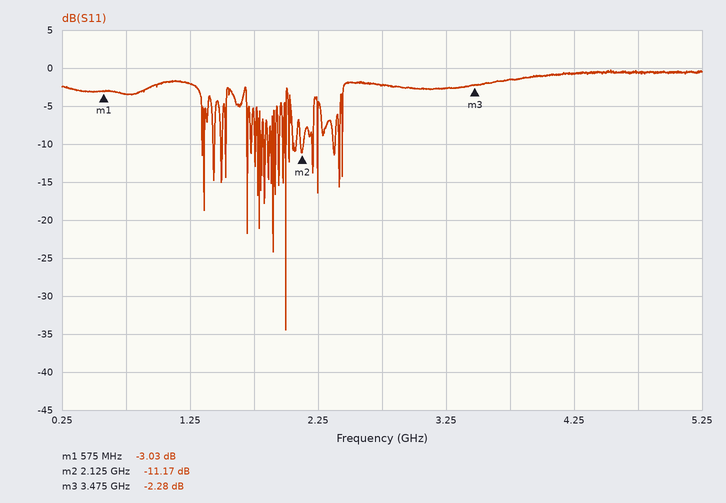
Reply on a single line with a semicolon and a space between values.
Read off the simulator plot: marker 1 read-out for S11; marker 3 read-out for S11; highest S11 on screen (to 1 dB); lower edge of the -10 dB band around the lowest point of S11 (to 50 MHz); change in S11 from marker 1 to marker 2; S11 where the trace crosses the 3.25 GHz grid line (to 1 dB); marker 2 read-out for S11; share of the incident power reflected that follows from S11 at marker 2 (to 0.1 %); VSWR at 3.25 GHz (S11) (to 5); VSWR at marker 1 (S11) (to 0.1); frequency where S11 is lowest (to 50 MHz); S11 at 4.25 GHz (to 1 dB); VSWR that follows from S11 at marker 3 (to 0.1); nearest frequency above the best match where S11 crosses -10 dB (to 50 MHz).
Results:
-3.03 dB; -2.28 dB; 0 dB; 2.00 GHz; -8.14 dB; -3 dB; -11.17 dB; 7.6 %; 5; 5.8; 2.00 GHz; -1 dB; 7.7; 2.00 GHz
